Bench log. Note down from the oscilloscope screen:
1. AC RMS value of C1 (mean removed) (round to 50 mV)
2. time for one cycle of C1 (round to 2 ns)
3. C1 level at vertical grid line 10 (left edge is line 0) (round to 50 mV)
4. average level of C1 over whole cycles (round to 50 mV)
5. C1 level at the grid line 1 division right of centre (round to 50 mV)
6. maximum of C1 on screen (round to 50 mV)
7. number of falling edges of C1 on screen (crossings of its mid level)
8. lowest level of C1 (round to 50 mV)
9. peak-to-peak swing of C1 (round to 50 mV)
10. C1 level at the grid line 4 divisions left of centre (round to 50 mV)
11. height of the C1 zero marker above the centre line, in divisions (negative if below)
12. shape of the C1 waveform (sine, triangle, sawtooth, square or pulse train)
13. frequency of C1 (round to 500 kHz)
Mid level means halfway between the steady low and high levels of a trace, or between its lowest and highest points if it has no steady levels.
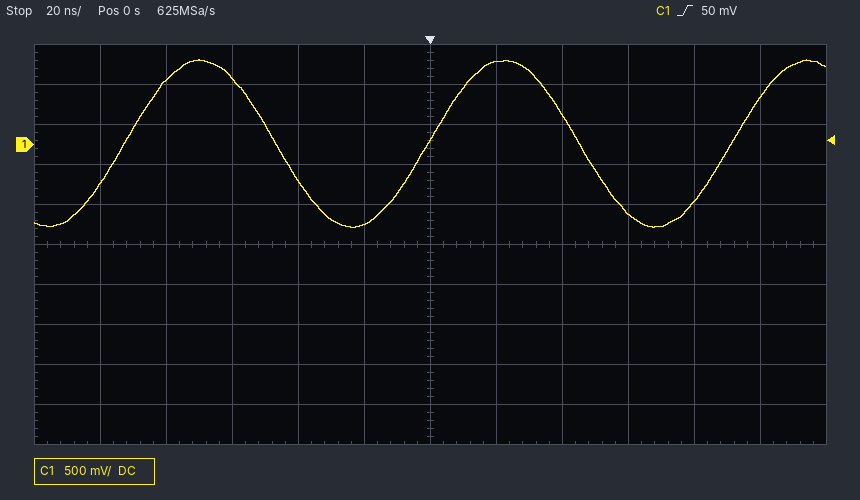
750 mV
92 ns
-700 mV
0 mV
1.05 V
1.05 V
2
-1.05 V
2.10 V
800 mV
+2.5 div
sine
11.0 MHz
